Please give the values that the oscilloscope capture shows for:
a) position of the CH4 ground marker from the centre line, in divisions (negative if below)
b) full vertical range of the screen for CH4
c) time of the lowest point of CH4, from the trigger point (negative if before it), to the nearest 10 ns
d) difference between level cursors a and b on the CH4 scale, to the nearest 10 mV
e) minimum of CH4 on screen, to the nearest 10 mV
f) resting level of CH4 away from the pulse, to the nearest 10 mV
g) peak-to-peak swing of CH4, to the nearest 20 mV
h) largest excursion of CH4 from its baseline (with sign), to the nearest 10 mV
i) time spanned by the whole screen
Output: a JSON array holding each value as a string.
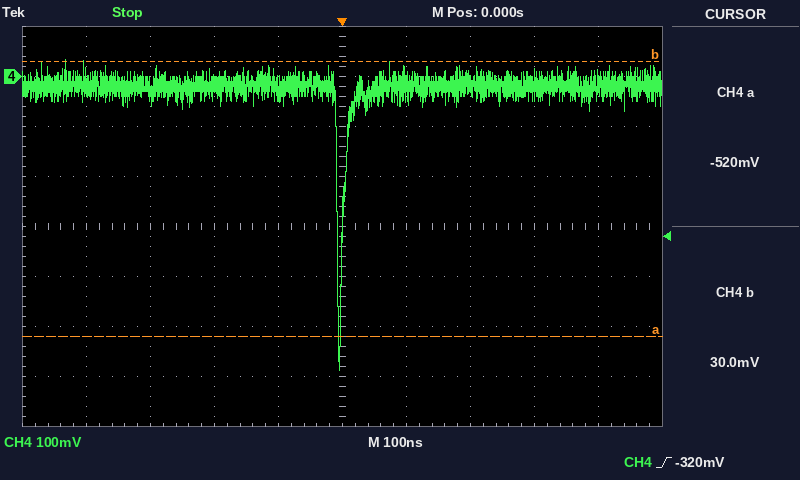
["+3.0 div", "800 mV", "0 ns", "550 mV", "-590 mV", "-20 mV", "620 mV", "-570 mV", "1 µs"]
